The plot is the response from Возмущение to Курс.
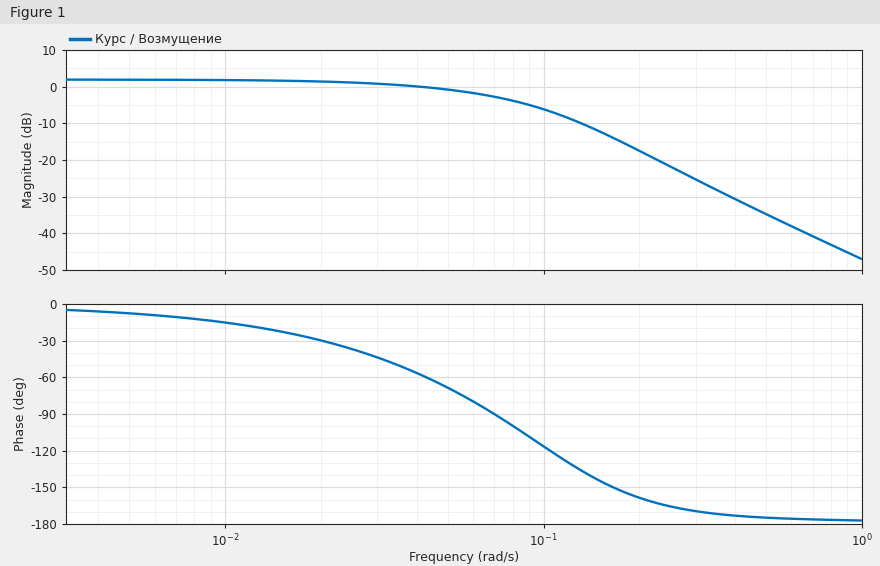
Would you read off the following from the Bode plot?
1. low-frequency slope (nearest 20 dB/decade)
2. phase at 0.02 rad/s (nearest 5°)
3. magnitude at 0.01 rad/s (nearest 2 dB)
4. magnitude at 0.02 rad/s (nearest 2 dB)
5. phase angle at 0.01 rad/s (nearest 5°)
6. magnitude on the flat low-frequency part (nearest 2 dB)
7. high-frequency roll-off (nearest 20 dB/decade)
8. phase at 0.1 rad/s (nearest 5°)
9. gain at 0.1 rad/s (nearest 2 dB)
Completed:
0 dB/decade
-30°
2 dB
2 dB
-15°
2 dB
-40 dB/decade
-115°
-6 dB
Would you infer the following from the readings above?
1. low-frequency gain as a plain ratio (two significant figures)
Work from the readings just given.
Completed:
1.3
